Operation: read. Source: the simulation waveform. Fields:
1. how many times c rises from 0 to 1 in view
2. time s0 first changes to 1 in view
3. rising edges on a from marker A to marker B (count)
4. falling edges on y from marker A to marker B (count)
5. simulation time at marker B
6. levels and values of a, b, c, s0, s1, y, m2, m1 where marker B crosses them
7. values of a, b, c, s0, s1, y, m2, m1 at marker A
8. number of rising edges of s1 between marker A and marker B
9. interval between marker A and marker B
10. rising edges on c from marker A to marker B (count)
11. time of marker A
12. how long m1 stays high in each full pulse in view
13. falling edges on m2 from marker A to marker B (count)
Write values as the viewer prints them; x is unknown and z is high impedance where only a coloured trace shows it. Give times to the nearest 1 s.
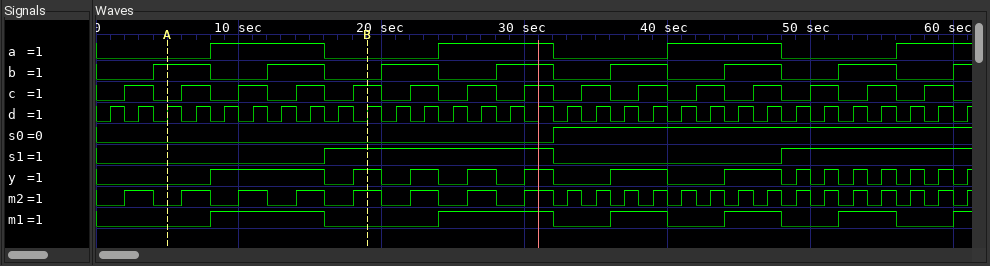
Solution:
15
32 s
1
1
19 s
a=0, b=0, c=1, s0=0, s1=1, y=1, m2=1, m1=0
a=0, b=1, c=0, s0=0, s1=0, y=0, m2=0, m1=0
1
14 s
4
5 s
8 s, 8 s, 4 s, 4 s, 4 s
3
